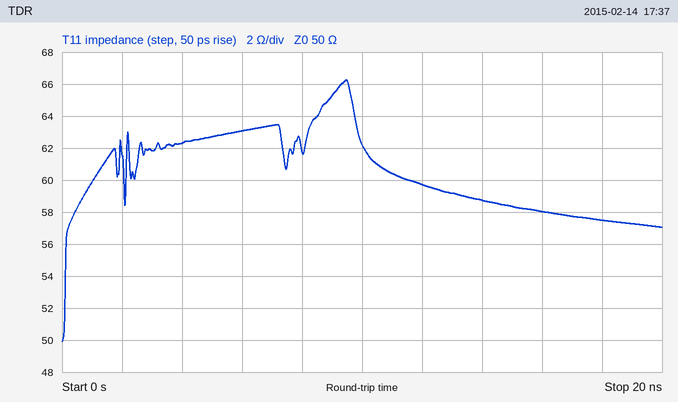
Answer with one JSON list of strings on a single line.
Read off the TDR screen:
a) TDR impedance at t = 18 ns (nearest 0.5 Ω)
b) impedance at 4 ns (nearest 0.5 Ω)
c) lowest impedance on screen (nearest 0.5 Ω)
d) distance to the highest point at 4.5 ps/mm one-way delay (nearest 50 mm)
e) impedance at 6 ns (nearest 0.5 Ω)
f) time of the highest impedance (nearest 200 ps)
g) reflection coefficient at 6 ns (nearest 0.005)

["57.5 Ω", "62.5 Ω", "50.0 Ω", "1.05 m", "63.0 Ω", "9.4 ns", "+0.115"]
